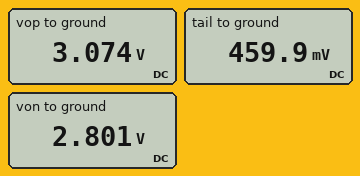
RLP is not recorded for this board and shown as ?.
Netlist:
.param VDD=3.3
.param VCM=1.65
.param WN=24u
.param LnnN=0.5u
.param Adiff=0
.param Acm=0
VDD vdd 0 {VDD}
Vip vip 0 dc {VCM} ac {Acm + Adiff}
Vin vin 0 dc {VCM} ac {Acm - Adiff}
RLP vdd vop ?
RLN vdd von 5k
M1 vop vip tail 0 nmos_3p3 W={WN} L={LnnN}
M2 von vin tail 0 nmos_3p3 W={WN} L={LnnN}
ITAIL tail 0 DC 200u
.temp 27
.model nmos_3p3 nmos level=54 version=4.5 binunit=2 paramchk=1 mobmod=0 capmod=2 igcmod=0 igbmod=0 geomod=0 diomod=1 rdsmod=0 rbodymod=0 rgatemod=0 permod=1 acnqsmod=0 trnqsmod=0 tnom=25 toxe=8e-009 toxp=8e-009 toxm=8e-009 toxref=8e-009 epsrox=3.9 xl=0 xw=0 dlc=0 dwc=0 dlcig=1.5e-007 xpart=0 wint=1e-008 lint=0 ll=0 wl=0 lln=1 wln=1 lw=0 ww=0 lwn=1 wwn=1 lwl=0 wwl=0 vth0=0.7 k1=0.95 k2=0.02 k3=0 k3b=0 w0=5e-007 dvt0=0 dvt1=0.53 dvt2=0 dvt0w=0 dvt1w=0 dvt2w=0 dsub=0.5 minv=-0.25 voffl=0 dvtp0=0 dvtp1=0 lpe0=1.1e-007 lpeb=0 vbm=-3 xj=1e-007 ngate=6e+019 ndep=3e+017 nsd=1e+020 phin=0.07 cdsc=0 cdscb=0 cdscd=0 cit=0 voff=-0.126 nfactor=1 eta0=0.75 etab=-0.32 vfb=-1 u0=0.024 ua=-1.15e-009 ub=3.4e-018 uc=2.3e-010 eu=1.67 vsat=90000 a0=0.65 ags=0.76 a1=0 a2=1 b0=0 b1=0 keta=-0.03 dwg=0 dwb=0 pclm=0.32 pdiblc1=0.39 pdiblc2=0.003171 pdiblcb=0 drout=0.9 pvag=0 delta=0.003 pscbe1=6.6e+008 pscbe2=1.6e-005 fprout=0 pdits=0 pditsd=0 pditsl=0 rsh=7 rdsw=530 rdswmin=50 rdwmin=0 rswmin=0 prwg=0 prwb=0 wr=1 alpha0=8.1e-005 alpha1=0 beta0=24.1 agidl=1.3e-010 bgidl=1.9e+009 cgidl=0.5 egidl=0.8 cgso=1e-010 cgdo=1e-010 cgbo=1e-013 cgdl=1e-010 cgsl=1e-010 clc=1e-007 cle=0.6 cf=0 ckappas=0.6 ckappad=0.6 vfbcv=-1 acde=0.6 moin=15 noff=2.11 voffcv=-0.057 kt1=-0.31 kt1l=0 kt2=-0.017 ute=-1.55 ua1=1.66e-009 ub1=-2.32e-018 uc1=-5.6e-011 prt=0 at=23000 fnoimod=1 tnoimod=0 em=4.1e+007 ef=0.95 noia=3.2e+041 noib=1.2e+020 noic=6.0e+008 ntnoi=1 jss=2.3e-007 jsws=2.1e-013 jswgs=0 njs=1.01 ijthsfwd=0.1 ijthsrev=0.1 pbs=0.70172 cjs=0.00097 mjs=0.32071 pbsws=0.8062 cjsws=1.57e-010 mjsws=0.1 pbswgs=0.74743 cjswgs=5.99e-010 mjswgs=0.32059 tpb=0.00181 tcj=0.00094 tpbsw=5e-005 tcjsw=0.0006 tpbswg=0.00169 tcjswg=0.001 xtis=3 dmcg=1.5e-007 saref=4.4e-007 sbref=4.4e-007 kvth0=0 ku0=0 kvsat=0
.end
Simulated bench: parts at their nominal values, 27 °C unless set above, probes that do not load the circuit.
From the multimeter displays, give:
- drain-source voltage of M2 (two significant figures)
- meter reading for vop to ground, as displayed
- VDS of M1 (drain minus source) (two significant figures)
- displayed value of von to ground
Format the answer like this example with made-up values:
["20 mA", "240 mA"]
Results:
["2.3 V", "3.074 V", "2.6 V", "2.801 V"]
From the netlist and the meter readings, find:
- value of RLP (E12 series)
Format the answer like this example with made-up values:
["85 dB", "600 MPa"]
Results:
["2.2 kΩ"]
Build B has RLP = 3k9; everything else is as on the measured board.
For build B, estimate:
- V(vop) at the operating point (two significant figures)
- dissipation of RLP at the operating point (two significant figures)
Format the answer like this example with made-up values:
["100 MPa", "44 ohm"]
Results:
["2.9 V", "40 µW"]
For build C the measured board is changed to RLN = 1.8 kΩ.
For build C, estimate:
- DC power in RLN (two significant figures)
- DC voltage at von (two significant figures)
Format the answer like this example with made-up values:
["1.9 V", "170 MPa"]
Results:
["19 µW", "3.1 V"]
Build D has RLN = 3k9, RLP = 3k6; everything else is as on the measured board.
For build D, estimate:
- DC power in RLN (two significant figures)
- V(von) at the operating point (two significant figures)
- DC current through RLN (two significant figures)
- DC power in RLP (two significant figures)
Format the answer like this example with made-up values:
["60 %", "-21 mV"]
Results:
["40 µW", "2.9 V", "100 µA", "37 µW"]
